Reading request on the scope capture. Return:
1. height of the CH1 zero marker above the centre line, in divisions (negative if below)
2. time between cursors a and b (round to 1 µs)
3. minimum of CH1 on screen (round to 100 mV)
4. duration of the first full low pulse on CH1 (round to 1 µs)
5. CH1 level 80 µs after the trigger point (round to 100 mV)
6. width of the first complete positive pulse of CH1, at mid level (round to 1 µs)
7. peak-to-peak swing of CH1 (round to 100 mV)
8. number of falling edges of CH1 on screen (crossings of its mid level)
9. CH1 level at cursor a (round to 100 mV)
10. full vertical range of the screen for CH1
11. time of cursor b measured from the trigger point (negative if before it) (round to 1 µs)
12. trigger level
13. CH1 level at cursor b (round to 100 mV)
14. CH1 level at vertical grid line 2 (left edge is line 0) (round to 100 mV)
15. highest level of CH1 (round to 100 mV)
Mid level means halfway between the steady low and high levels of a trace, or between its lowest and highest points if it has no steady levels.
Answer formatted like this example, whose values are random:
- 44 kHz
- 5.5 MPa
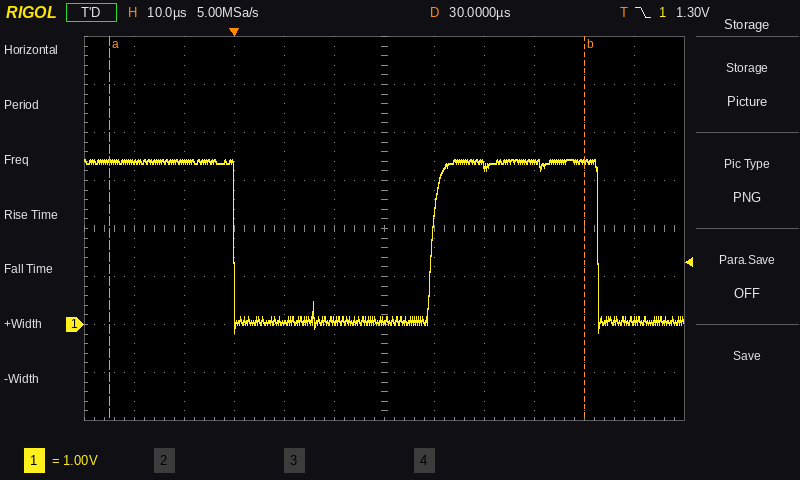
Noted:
- -2.0 div
- 95 µs
- -200 mV
- 40 µs
- 100 mV
- 33 µs
- 3.6 V
- 2
- 3.4 V
- 8 V
- +70 µs
- 1.30 V
- 3.4 V
- 3.4 V
- 3.4 V
